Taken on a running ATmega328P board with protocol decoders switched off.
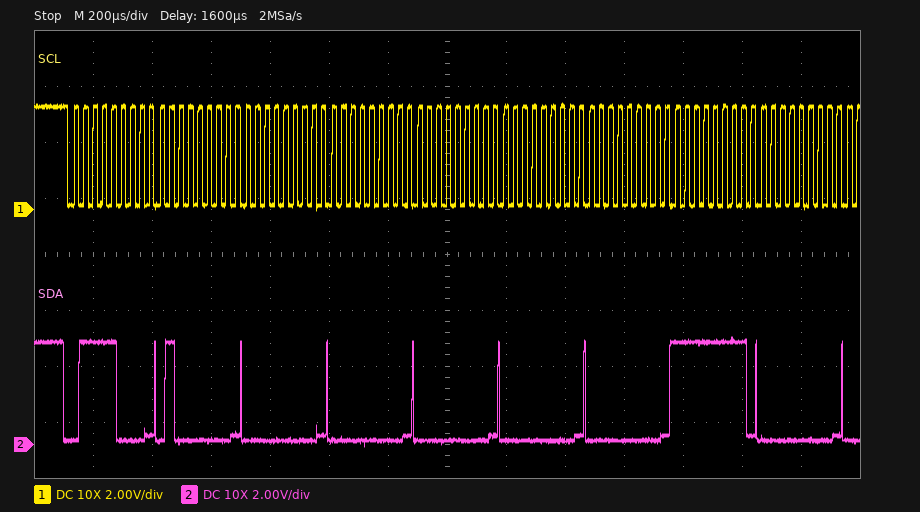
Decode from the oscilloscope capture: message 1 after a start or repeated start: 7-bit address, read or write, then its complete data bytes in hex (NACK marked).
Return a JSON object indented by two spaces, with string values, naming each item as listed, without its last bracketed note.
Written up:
{
  "message 1 after a start or repeated start: 7-bit address, read or write, then its complete data bytes in hex": "0x3C write: 40 00 00 00 00 00 FF 00"
}
